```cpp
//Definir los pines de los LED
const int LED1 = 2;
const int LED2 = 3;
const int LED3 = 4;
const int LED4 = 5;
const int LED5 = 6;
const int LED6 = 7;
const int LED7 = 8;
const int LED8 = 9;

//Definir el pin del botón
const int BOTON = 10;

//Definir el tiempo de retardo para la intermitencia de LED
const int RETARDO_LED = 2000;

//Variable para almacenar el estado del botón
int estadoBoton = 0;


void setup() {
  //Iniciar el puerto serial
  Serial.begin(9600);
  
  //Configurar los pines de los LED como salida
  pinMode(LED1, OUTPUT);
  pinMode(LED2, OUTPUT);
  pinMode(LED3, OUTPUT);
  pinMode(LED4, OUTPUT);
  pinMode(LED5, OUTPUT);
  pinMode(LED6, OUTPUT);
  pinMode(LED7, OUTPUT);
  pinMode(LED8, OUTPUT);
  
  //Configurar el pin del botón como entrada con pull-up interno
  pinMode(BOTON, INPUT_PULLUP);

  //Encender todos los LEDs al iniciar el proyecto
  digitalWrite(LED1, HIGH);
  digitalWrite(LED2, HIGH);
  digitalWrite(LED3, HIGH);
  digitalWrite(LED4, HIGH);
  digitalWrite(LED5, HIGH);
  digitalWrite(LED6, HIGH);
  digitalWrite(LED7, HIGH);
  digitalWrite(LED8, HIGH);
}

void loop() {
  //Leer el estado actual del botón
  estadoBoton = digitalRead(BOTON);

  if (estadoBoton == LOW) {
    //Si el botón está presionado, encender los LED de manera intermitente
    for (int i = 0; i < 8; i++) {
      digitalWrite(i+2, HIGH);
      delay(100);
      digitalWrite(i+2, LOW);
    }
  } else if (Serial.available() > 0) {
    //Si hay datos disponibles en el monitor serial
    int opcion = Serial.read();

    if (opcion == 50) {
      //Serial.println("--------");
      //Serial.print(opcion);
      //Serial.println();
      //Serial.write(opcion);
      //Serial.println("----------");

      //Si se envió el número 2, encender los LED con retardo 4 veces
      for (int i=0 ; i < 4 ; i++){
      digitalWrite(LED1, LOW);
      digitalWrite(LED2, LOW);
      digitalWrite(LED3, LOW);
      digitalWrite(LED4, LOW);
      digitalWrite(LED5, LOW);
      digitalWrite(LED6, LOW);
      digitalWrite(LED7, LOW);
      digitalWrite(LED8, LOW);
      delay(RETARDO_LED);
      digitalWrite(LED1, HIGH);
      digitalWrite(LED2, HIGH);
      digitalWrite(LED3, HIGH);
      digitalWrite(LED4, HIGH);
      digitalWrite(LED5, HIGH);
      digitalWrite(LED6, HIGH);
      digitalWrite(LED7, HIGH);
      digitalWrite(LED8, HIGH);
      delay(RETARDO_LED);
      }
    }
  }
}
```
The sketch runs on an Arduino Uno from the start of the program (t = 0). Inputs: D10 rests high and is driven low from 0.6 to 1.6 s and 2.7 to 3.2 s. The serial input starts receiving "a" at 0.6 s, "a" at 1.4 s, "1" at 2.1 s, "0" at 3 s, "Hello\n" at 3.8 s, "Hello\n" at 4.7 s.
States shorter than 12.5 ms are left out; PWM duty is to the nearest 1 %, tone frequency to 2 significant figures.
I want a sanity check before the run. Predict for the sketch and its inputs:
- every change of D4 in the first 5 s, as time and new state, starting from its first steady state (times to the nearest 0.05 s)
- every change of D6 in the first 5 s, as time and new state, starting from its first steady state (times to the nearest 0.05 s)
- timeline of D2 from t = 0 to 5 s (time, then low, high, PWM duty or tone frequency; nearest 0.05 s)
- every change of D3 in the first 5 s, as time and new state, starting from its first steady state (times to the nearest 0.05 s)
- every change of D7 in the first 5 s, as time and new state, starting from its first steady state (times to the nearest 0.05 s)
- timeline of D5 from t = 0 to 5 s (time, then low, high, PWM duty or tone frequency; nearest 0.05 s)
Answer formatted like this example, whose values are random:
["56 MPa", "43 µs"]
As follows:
["0 s high; 0.9 s low; 1.6 s high; 1.7 s low; 2.9 s high; 3 s low", "0 s high; 1.1 s low; 1.8 s high; 1.9 s low; 3.1 s high; 3.2 s low", "0 s high; 0.7 s low; 1.4 s high; 1.5 s low; 2.7 s high; 2.8 s low", "0 s high; 0.8 s low; 1.5 s high; 1.6 s low; 2.8 s high; 2.9 s low", "0 s high; 1.2 s low; 1.9 s high; 2 s low; 3.2 s high; 3.3 s low", "0 s high; 1 s low; 1.7 s high; 1.8 s low; 3 s high; 3.1 s low"]
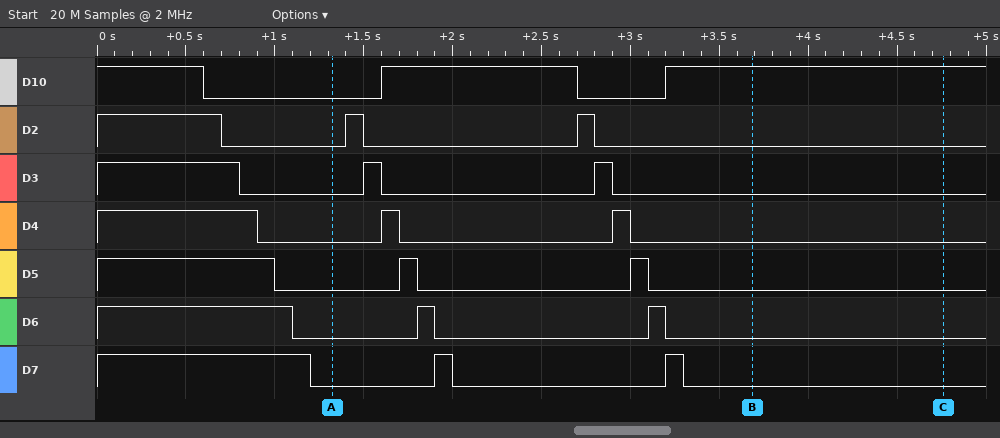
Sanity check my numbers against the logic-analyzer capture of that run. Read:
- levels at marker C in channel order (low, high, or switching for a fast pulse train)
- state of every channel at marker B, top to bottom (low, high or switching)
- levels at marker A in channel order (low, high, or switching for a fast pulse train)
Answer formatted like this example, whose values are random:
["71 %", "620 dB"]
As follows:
["D10 high, D2 low, D3 low, D4 low, D5 low, D6 low, D7 low", "D10 high, D2 low, D3 low, D4 low, D5 low, D6 low, D7 low", "D10 low, D2 low, D3 low, D4 low, D5 low, D6 low, D7 low"]
